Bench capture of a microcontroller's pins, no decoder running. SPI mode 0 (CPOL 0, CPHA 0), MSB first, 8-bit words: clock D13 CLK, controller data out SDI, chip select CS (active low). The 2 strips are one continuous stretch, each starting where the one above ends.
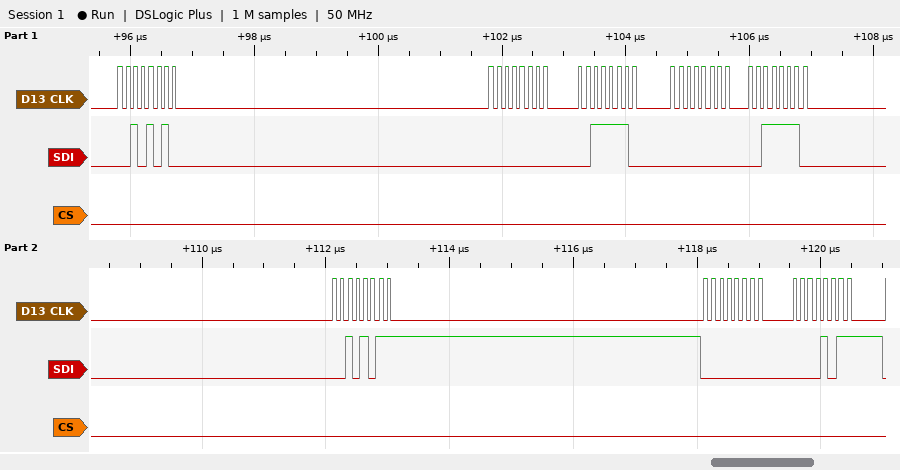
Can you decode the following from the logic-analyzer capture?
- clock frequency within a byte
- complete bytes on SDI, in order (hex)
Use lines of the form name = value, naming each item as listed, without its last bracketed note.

clock frequency within a byte = 8 MHz
complete bytes on SDI, in order = 2A 00 3E 00 3E 2B 00 0B
